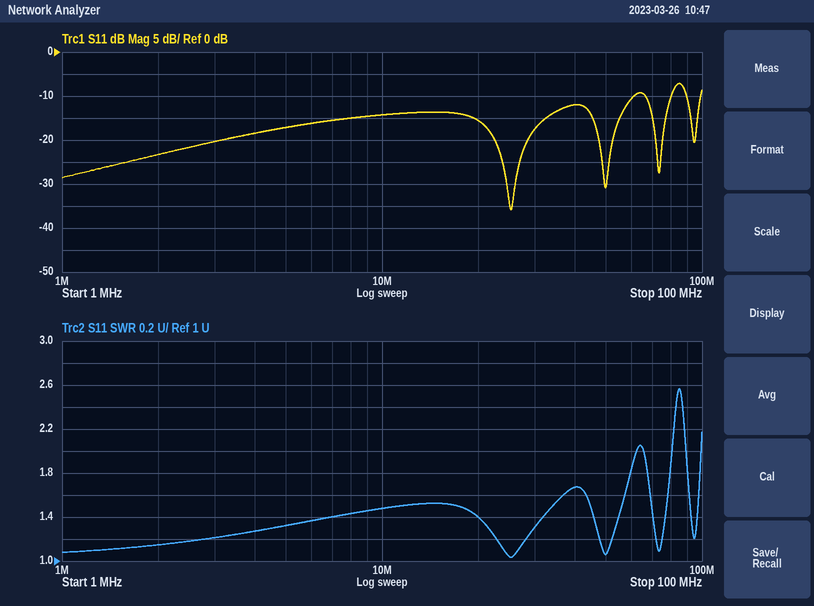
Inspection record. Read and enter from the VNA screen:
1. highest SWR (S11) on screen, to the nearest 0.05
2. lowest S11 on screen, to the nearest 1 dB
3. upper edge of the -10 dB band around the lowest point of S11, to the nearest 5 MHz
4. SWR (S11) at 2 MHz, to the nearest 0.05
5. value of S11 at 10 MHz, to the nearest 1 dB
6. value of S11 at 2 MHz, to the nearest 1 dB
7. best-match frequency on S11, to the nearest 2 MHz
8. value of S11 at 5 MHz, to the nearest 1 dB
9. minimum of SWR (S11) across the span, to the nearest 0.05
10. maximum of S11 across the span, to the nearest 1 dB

2.55
-36 dB
60 MHz
1.15
-14 dB
-23 dB
26 MHz
-17 dB
1.05
-7 dB
